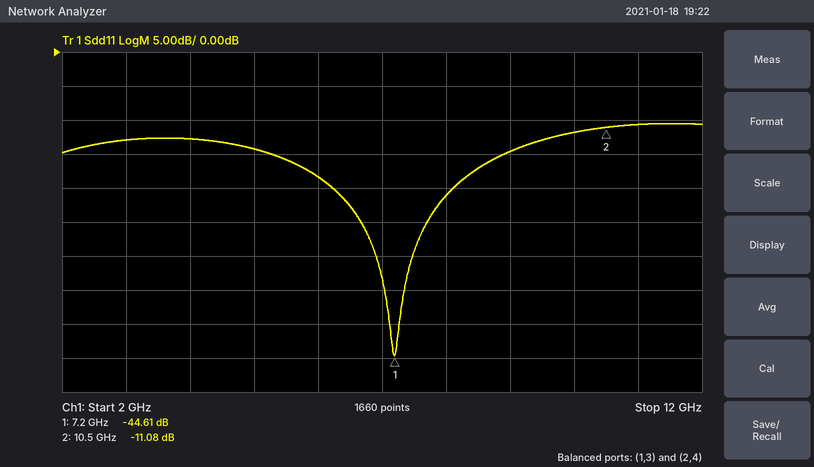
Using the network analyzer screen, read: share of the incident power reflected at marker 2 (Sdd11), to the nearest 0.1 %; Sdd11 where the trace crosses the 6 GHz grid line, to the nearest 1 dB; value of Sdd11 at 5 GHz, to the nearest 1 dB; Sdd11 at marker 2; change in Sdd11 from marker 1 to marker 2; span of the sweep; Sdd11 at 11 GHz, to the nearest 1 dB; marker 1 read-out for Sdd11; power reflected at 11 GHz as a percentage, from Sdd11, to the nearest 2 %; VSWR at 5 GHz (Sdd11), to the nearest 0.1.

7.8 %
-18 dB
-14 dB
-11.08 dB
33.53 dB
10 GHz
-11 dB
-44.61 dB
8 %
1.5
